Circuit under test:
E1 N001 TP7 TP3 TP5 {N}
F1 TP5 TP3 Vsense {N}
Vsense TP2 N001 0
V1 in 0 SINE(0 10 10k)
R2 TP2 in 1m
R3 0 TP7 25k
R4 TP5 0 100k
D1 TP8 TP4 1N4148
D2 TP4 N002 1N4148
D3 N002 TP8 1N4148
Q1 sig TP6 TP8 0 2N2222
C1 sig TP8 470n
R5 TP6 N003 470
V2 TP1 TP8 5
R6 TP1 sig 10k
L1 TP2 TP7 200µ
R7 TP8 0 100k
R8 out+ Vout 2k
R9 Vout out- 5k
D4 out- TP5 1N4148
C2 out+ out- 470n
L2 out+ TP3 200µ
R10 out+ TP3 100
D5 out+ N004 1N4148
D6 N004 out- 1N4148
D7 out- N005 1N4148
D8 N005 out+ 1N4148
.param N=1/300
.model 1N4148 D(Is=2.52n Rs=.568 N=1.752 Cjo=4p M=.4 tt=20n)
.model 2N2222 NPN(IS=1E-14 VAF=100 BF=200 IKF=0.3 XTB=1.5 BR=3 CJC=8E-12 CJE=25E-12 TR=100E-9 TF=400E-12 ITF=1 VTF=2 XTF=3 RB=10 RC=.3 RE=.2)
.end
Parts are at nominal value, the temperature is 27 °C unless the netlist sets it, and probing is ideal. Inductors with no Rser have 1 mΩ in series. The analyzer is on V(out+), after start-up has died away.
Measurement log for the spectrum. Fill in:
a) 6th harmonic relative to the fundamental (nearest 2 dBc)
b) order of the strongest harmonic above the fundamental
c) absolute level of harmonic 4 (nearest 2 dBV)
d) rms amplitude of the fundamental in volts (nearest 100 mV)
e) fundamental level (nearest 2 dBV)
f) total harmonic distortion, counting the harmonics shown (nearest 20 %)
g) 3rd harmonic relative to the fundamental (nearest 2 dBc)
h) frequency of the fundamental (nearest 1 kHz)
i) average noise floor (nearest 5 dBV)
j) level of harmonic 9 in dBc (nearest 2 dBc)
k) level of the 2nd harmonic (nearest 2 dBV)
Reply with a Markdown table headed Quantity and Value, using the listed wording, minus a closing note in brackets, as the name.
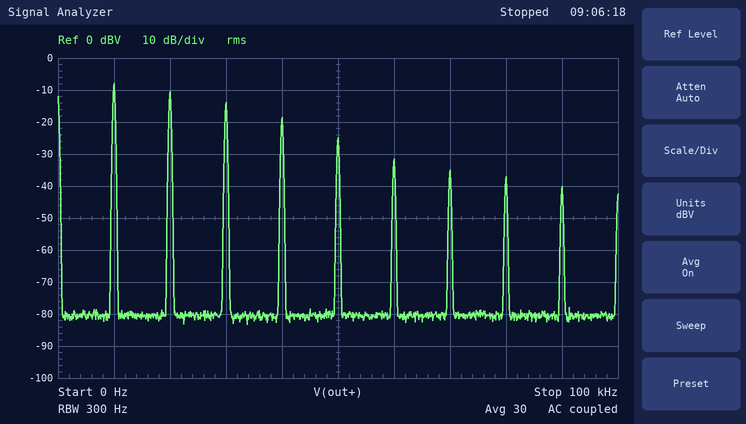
| Quantity | Value |
|---|---|
| 6th harmonic relative to the fundamental | -24 dBc |
| order of the strongest harmonic above the fundamental | 2 |
| absolute level of harmonic 4 | -18 dBV |
| rms amplitude of the fundamental in volts | 400 mV |
| fundamental level | -8 dBV |
| total harmonic distortion, counting the harmonics shown | 100 % |
| 3rd harmonic relative to the fundamental | -6 dBc |
| frequency of the fundamental | 10 kHz |
| average noise floor | -80 dBV |
| level of harmonic 9 in dBc | -32 dBc |
| level of the 2nd harmonic | -10 dBV |
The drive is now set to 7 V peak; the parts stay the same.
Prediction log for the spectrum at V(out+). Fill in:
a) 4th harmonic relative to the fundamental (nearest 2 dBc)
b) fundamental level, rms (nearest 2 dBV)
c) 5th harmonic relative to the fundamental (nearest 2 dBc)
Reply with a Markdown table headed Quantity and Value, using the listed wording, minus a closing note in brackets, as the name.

| Quantity | Value |
|---|---|
| 4th harmonic relative to the fundamental | -12 dBc |
| fundamental level, rms | -8 dBV |
| 5th harmonic relative to the fundamental | -20 dBc |
